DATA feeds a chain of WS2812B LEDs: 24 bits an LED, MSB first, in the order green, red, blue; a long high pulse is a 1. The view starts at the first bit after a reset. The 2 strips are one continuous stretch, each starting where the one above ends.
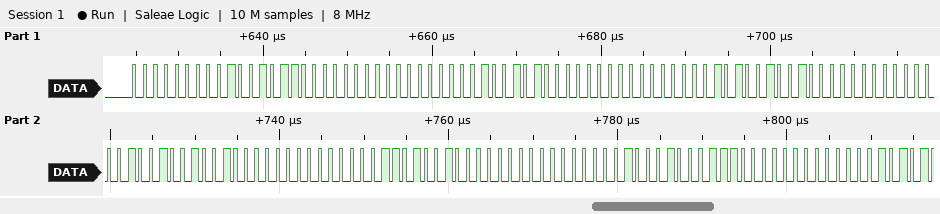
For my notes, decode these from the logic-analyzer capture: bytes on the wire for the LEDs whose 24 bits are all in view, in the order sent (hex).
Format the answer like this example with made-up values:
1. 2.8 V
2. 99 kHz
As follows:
1. 00 4B 00 00 4A 00 01 49 00 02 49 00 03 48 00 04 47 00
